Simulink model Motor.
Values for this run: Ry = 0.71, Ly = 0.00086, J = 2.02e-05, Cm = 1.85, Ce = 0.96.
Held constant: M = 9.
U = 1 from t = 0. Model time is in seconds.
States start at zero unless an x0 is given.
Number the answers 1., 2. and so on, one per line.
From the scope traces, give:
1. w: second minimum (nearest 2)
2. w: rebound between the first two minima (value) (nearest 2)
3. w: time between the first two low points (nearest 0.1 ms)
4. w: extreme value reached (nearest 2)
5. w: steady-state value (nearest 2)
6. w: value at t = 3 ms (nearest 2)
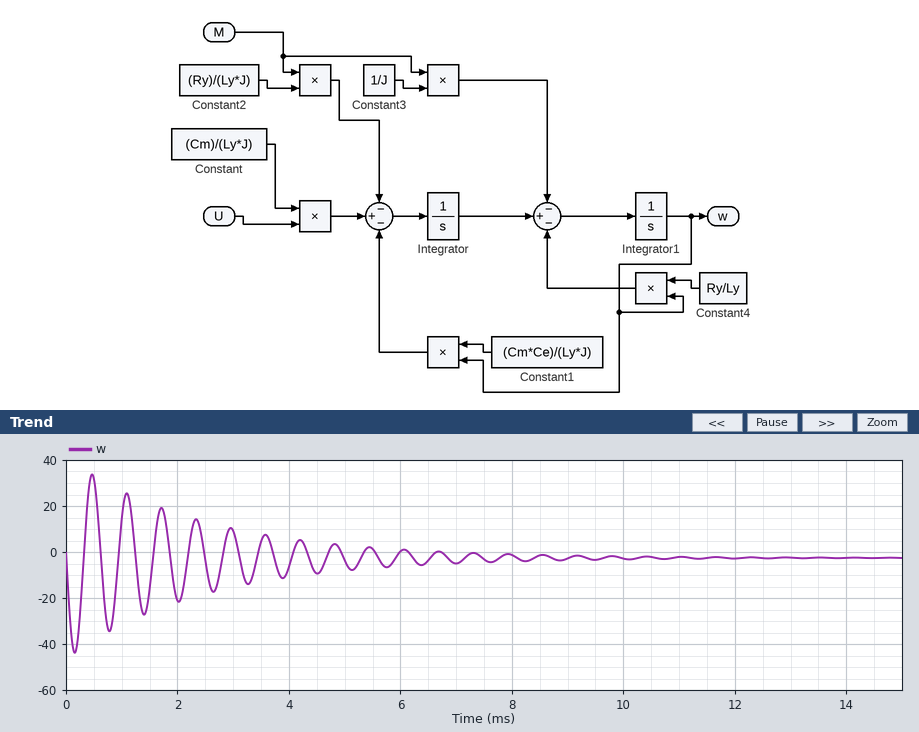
1. -34
2. 34
3. 0.6 ms
4. -44
5. -2
6. 10
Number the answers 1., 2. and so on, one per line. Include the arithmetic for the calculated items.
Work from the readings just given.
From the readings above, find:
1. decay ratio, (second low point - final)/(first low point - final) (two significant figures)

1. (-34 - (-2)) / (-44 - (-2)) = 0.76
